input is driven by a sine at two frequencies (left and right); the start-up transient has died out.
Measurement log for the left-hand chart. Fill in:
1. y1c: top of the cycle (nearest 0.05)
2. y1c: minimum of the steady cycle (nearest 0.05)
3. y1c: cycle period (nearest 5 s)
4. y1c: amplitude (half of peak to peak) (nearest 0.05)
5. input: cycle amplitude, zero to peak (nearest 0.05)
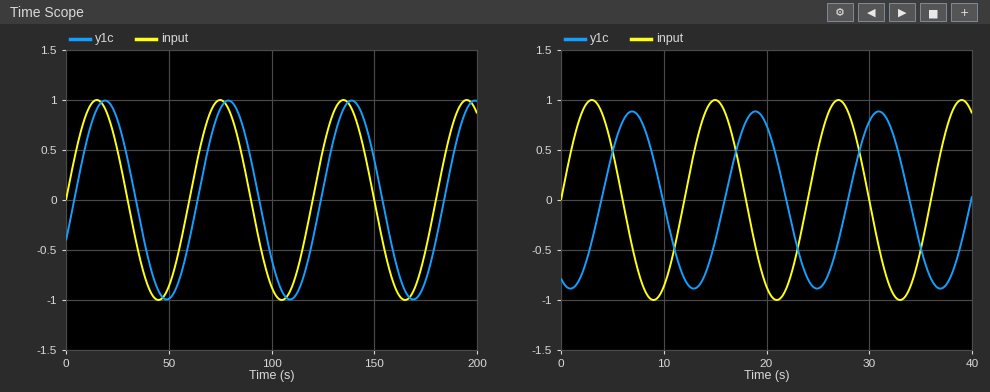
1.00
-1.00
60 s
1.00
1.00
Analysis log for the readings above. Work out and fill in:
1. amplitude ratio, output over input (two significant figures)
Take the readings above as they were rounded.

1.0
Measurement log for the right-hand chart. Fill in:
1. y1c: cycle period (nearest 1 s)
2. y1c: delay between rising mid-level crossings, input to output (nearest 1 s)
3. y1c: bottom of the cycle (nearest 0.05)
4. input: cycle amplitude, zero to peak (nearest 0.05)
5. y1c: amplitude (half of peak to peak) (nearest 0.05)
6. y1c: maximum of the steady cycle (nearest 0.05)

12 s
4 s
-0.90
1.00
0.90
0.90
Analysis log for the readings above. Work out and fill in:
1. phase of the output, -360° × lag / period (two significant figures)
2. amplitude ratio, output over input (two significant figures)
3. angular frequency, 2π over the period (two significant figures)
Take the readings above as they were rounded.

-120°
0.90
0.52 rad/s
